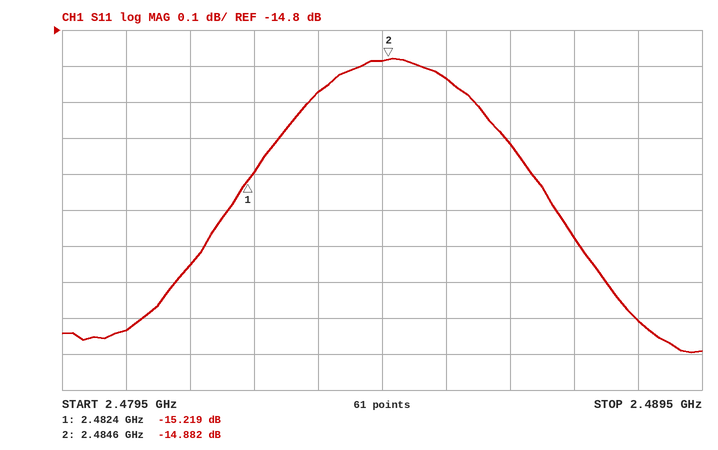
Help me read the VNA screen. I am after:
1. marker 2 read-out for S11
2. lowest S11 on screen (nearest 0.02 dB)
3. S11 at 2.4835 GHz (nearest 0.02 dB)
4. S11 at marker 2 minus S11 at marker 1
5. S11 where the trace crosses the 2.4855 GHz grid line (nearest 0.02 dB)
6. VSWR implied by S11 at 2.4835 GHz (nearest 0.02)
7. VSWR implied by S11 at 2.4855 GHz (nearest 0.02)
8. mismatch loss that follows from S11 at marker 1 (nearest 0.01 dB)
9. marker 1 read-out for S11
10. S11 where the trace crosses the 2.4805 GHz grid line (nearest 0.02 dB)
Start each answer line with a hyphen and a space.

- -14.882 dB
- -15.70 dB
- -14.98 dB
- 0.337 dB
- -14.94 dB
- 1.44
- 1.44
- 0.13 dB
- -15.219 dB
- -15.64 dB
